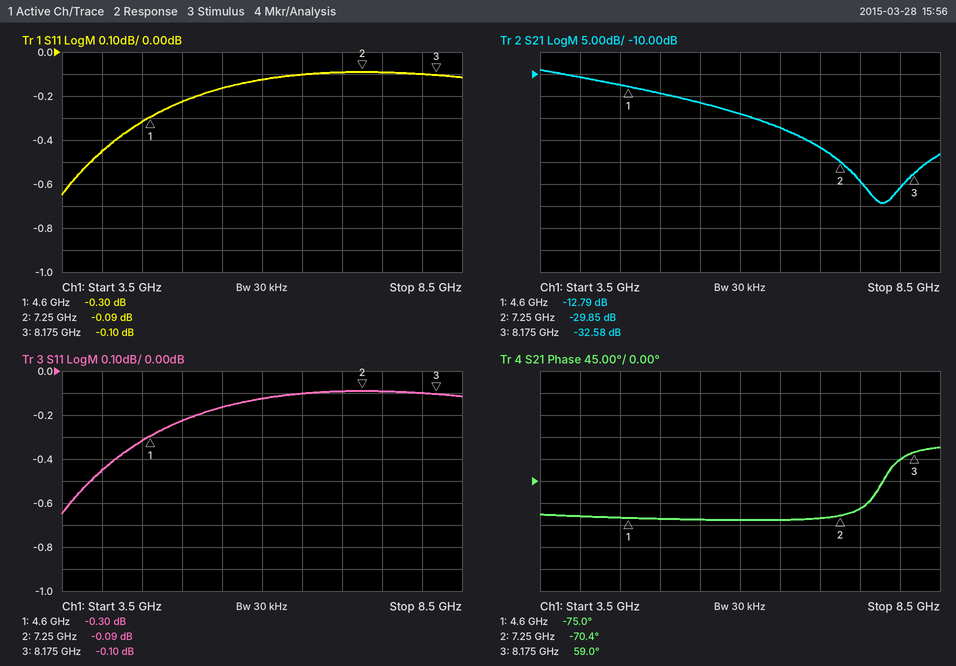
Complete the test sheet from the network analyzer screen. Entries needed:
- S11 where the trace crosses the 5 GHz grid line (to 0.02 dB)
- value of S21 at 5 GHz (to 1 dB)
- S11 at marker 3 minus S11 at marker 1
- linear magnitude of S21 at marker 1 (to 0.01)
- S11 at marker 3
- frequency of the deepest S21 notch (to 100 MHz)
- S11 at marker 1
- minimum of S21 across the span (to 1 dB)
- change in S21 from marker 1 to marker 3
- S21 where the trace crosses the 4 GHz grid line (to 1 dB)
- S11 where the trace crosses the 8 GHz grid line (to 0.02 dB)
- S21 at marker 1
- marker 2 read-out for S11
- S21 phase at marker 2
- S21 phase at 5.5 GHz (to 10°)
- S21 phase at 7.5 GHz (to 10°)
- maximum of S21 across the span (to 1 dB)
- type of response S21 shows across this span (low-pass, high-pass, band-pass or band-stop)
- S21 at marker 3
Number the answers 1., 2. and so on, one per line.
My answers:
1. -0.22 dB
2. -14 dB
3. 0.20 dB
4. 0.23
5. -0.10 dB
6. 7.8 GHz
7. -0.30 dB
8. -39 dB
9. -19.79 dB
10. -11 dB
11. -0.10 dB
12. -12.79 dB
13. -0.09 dB
14. -70.4°
15. -80°
16. -60°
17. -9 dB
18. low-pass
19. -32.58 dB
